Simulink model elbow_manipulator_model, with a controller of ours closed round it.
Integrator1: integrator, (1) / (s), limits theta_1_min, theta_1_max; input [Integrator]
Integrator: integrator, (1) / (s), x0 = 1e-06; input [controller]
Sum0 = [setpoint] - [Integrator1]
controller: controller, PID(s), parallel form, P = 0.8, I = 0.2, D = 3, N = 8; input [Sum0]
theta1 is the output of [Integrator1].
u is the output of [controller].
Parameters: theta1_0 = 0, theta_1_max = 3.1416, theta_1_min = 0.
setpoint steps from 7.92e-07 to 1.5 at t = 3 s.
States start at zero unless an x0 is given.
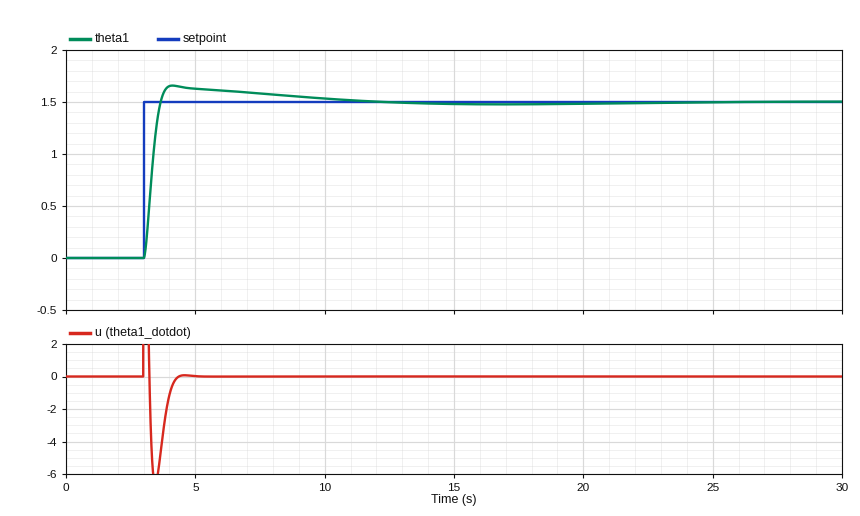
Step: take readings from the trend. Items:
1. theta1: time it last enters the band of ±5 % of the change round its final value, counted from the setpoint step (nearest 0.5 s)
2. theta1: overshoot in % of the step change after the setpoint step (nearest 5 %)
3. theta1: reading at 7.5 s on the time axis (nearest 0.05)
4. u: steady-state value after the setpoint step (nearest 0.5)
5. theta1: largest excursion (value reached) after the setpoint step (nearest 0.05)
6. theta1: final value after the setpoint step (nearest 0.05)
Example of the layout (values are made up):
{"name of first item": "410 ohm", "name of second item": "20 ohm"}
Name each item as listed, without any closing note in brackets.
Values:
{"theta1: time it last enters the band of ±5 % of the change round its final value, counted from the setpoint step": "5.0 s", "theta1: overshoot in % of the step change after the setpoint step": "10 %", "theta1: reading at 7.5 s on the time axis": "1.60", "u: steady-state value after the setpoint step": "0.0", "theta1: largest excursion (value reached) after the setpoint step": "1.65", "theta1: final value after the setpoint step": "1.50"}
